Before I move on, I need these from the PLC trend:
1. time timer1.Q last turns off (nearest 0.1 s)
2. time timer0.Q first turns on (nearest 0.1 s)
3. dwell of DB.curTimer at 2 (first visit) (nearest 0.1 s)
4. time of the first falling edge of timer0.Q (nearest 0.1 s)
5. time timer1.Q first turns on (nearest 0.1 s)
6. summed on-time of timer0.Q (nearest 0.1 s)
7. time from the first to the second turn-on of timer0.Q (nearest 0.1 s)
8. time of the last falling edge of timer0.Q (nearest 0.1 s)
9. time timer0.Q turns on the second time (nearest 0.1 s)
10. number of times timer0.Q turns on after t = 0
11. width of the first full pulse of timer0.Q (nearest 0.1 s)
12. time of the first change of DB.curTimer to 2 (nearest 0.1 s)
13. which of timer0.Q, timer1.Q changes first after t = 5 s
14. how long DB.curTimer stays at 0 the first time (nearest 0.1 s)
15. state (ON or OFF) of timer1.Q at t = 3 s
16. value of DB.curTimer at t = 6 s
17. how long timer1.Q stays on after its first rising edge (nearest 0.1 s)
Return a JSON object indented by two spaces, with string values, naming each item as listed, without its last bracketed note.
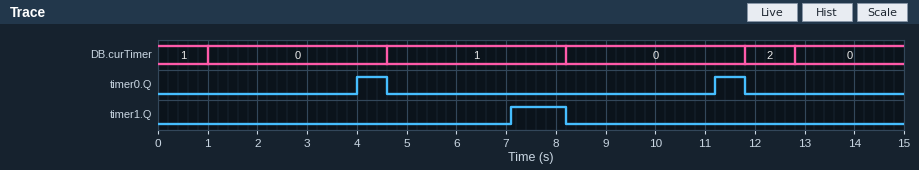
{
  "time timer1.Q last turns off": "8.2 s",
  "time timer0.Q first turns on": "4.0 s",
  "dwell of DB.curTimer at 2 (first visit)": "1.0 s",
  "time of the first falling edge of timer0.Q": "4.6 s",
  "time timer1.Q first turns on": "7.1 s",
  "summed on-time of timer0.Q": "1.2 s",
  "time from the first to the second turn-on of timer0.Q": "7.2 s",
  "time of the last falling edge of timer0.Q": "11.8 s",
  "time timer0.Q turns on the second time": "11.2 s",
  "number of times timer0.Q turns on after t = 0": "2",
  "width of the first full pulse of timer0.Q": "0.6 s",
  "time of the first change of DB.curTimer to 2": "11.8 s",
  "which of timer0.Q, timer1.Q changes first after t = 5 s": "timer1.Q",
  "how long DB.curTimer stays at 0 the first time": "3.6 s",
  "state (ON or OFF) of timer1.Q at t = 3 s": "OFF",
  "value of DB.curTimer at t = 6 s": "1",
  "how long timer1.Q stays on after its first rising edge": "1.1 s"
}
